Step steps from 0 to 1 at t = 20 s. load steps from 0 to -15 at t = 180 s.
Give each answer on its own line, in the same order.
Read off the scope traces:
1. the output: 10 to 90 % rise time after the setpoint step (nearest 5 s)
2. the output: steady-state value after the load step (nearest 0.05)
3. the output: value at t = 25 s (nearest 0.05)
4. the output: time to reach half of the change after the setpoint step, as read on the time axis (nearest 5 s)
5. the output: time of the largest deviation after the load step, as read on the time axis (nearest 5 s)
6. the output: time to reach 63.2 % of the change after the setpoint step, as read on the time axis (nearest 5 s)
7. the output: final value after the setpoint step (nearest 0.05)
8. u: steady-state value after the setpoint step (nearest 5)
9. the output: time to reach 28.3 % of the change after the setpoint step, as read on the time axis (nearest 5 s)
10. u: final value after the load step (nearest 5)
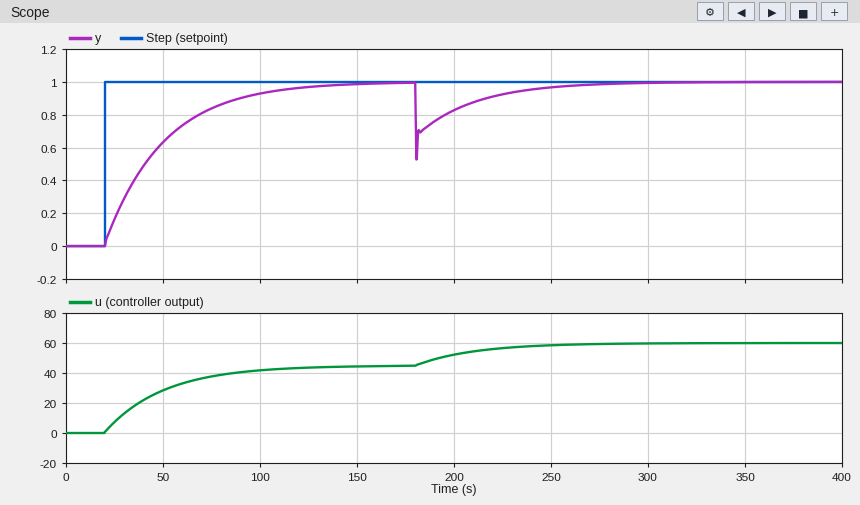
65 s
1.00
0.15
40 s
180 s
50 s
1.00
45
30 s
60
